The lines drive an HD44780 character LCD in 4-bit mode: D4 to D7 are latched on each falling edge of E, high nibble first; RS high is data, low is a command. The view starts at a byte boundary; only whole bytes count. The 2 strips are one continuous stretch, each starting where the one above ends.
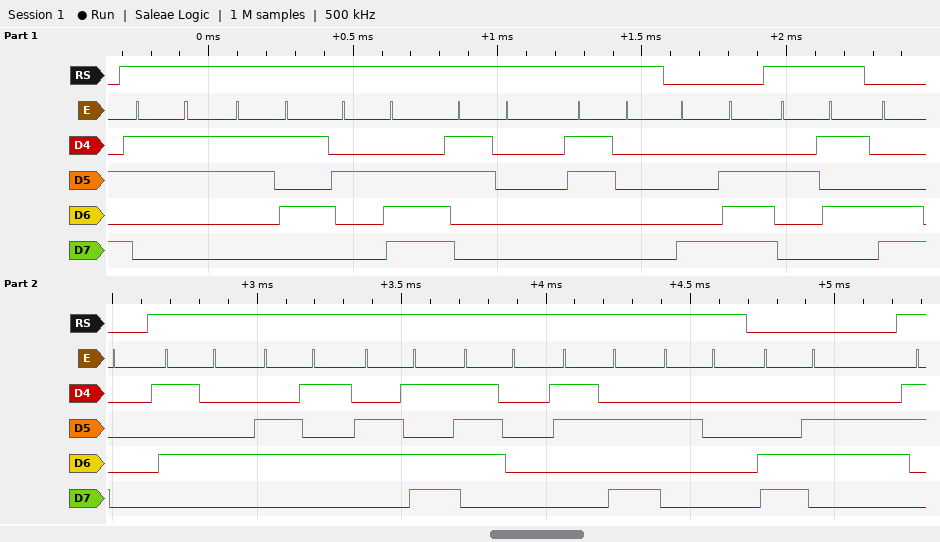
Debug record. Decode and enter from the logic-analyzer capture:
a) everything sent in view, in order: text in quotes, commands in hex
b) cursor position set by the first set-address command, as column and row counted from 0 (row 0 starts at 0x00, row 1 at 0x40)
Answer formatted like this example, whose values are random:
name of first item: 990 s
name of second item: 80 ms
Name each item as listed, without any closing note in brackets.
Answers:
everything sent in view, in order: text in quotes, commands in hex: "35.00" 0x8E "%" 0xC0 "Temp: " 0xC6
cursor position set by the first set-address command, as column and row counted from 0: column 14, row 0
